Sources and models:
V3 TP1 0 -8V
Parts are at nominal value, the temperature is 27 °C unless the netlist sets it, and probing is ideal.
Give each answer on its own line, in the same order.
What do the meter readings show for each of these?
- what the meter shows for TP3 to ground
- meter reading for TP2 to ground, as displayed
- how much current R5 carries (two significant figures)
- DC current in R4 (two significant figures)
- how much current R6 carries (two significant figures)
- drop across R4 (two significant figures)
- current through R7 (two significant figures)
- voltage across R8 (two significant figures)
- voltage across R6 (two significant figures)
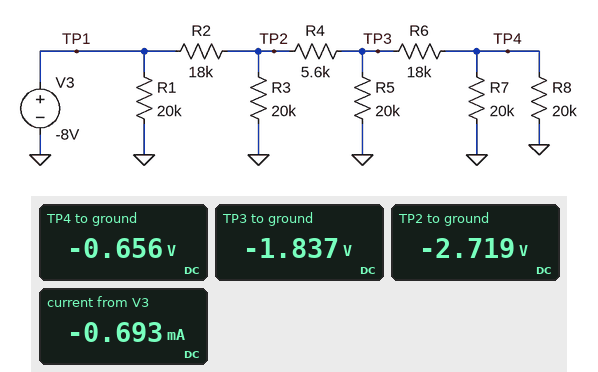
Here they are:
-1.837 V
-2.719 V
92 µA
160 µA
66 µA
880 mV
33 µA
660 mV
1.2 V
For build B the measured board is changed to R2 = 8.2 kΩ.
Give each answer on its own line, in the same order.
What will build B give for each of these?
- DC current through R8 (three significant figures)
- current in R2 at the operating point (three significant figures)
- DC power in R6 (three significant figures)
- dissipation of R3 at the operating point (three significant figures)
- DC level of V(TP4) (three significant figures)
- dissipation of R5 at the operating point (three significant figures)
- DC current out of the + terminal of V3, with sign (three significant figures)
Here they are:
51.2 µA
458 µA
189 µW
901 µW
-1.02 V
411 µW
-858 µA
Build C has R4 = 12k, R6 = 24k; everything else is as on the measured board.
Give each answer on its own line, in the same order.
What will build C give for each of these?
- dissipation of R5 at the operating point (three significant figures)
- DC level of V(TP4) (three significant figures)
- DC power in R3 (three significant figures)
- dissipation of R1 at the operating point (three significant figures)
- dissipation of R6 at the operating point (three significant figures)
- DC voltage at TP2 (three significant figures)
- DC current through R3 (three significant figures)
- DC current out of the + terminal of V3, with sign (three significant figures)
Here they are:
121 µW
-458 mV
462 µW
3.20 mW
50.3 µW
-3.04 V
152 µA
-676 µA
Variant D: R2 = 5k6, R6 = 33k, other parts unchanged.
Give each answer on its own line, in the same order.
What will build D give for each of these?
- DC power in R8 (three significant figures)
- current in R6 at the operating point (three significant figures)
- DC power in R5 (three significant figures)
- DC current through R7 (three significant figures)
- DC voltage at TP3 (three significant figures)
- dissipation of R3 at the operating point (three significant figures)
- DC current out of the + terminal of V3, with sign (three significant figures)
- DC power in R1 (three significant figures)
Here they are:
35.3 µW
84.0 µA
652 µW
42.0 µA
-3.61 V
1.30 mW
-919 µA
3.20 mW
